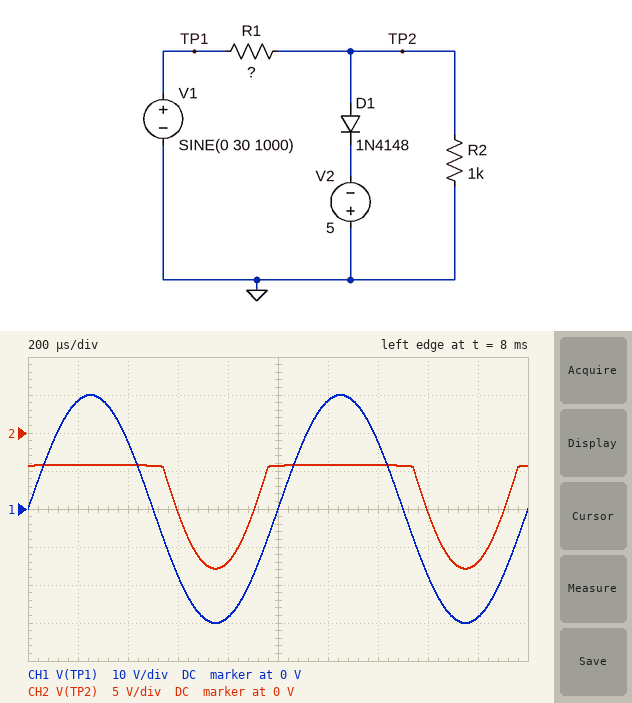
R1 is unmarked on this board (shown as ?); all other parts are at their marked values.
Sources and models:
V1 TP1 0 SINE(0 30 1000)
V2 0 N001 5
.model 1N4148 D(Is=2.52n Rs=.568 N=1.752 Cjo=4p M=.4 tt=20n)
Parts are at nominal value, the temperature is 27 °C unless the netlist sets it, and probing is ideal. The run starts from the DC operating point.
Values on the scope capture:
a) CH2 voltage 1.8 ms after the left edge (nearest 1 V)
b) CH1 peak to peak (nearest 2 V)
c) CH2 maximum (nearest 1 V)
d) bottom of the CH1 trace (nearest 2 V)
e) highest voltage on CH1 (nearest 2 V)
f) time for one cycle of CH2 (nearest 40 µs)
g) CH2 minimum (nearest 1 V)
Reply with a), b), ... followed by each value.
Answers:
a) -17 V
b) 60 V
c) -4 V
d) -30 V
e) 30 V
f) 1.00 ms
g) -18 V
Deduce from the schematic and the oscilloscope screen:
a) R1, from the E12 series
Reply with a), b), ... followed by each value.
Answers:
a) 680 Ω
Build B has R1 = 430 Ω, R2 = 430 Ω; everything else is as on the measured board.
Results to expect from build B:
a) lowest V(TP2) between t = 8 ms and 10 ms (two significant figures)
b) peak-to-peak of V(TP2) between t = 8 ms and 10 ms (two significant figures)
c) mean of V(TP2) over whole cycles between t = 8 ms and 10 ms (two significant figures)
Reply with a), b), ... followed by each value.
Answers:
a) -15 V
b) 11 V
c) -7.1 V
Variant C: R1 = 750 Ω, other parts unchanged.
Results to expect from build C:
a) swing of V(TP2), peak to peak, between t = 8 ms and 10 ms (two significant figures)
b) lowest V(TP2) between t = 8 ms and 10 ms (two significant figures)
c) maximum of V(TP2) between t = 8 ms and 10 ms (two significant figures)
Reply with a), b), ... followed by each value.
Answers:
a) 13 V
b) -17 V
c) -4.2 V
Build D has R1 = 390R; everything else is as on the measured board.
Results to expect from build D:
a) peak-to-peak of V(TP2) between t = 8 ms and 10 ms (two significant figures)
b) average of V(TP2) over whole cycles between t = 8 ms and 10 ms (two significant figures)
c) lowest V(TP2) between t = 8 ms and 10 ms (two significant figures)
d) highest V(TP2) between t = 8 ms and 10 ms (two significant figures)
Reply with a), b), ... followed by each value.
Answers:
a) 17 V
b) -9.1 V
c) -22 V
d) -4.2 V
